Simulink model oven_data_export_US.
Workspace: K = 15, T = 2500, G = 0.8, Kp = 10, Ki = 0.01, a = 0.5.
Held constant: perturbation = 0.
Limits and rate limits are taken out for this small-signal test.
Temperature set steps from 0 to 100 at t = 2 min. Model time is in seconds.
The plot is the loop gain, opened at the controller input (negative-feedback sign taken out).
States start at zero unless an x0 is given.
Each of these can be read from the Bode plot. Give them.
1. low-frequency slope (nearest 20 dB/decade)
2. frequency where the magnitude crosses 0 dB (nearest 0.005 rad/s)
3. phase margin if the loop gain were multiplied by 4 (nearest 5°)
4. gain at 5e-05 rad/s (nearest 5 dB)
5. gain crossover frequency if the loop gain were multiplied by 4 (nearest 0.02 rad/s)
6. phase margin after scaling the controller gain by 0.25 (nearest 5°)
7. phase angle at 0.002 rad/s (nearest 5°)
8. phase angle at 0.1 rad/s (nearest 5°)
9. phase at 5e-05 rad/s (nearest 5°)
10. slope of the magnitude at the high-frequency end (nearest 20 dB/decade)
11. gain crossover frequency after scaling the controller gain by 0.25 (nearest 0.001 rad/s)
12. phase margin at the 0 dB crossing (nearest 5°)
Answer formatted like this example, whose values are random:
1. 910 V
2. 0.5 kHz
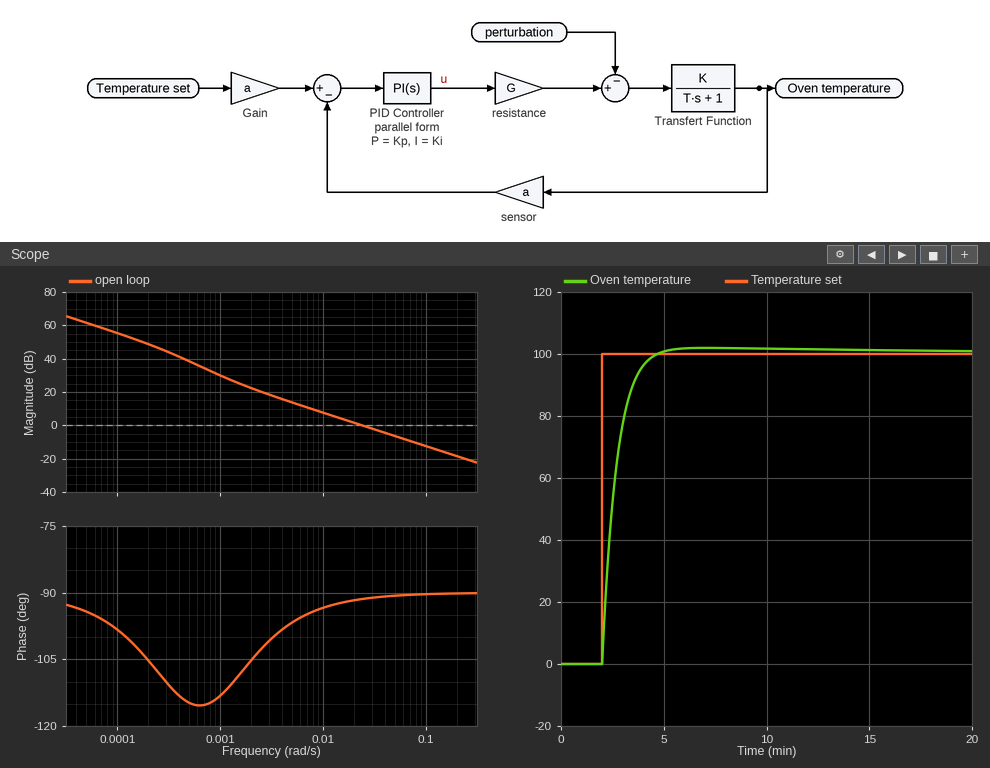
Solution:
1. -20 dB/decade
2. 0.025 rad/s
3. 90°
4. 60 dB
5. 0.10 rad/s
6. 85°
7. -105°
8. -90°
9. -95°
10. -20 dB/decade
11. 0.006 rad/s
12. 90°
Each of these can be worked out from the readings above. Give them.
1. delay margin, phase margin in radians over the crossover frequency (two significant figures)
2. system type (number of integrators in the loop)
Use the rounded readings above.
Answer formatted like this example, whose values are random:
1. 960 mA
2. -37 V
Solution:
1. 63 s
2. 1
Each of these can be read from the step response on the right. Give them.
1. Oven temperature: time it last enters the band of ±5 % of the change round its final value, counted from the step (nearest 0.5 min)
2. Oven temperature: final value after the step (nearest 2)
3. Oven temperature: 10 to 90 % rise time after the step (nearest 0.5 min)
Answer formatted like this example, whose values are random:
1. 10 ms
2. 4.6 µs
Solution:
1. 2.0 min
2. 100
3. 1.5 min
